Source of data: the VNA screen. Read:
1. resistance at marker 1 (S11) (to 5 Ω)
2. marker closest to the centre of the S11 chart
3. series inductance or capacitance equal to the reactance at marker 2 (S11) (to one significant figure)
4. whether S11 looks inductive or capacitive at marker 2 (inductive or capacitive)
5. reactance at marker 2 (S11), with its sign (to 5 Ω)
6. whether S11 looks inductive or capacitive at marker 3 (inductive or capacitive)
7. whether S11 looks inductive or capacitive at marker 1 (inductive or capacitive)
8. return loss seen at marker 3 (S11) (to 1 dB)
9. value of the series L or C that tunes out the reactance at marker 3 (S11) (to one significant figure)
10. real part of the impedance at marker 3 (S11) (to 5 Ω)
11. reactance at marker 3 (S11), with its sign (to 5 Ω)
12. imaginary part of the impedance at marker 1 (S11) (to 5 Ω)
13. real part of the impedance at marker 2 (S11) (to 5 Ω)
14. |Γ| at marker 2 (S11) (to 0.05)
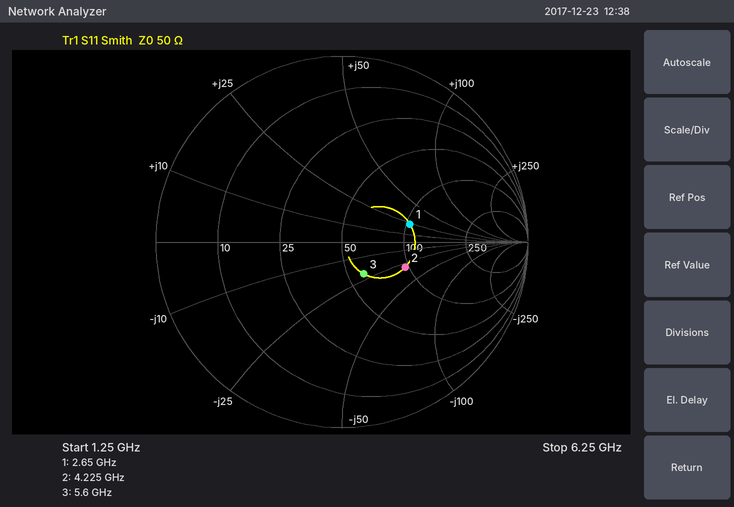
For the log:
105 Ω
marker 3
1 pF
capacitive
-30 Ω
capacitive
inductive
14 dB
600 pH
60 Ω
-20 Ω
+25 Ω
95 Ω
0.35
